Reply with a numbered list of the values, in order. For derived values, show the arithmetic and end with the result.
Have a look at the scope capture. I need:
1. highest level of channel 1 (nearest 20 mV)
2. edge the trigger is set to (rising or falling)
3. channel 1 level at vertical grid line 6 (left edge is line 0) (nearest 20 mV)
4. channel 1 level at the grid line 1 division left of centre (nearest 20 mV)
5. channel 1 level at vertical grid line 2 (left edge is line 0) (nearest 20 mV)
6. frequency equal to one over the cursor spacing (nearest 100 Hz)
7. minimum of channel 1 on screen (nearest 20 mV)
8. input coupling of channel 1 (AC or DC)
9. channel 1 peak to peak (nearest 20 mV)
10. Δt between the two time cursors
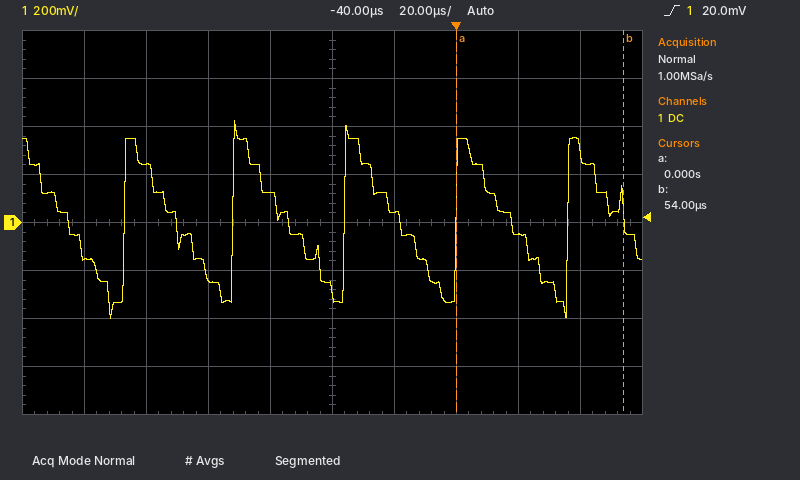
1. 420 mV
2. rising
3. 40 mV
4. 120 mV
5. 240 mV
6. 1 / 54 µs ≈ 18.5 kHz
7. -400 mV
8. DC
9. 420 mV − (-400 mV) = 820 mV
10. 54 µs − (0 s) = 54 µs
